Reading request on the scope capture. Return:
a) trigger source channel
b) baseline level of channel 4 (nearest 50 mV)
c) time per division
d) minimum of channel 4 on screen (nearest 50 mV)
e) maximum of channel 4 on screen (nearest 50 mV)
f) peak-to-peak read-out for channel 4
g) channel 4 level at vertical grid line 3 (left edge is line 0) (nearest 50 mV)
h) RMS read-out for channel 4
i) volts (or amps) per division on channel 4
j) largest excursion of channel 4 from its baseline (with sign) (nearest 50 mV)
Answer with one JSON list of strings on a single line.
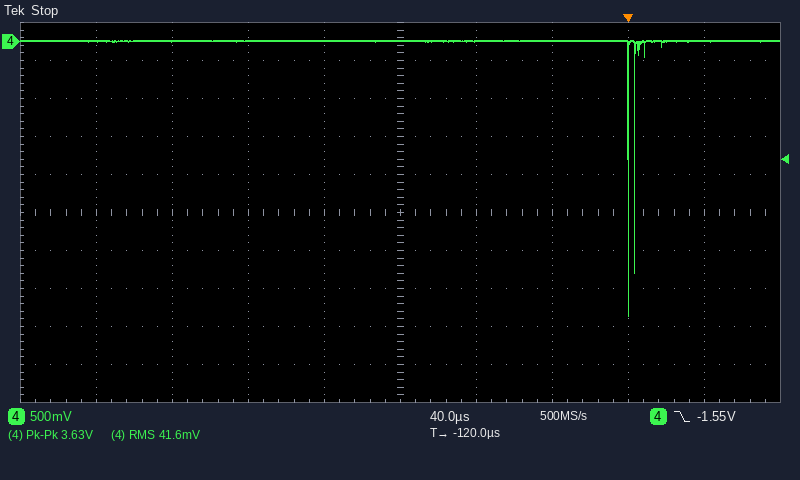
["channel 4", "0 mV", "40 µs", "-3.60 V", "0 mV", "3.63 V", "0 mV", "41.6 mV", "500 mV", "-3.60 V"]
